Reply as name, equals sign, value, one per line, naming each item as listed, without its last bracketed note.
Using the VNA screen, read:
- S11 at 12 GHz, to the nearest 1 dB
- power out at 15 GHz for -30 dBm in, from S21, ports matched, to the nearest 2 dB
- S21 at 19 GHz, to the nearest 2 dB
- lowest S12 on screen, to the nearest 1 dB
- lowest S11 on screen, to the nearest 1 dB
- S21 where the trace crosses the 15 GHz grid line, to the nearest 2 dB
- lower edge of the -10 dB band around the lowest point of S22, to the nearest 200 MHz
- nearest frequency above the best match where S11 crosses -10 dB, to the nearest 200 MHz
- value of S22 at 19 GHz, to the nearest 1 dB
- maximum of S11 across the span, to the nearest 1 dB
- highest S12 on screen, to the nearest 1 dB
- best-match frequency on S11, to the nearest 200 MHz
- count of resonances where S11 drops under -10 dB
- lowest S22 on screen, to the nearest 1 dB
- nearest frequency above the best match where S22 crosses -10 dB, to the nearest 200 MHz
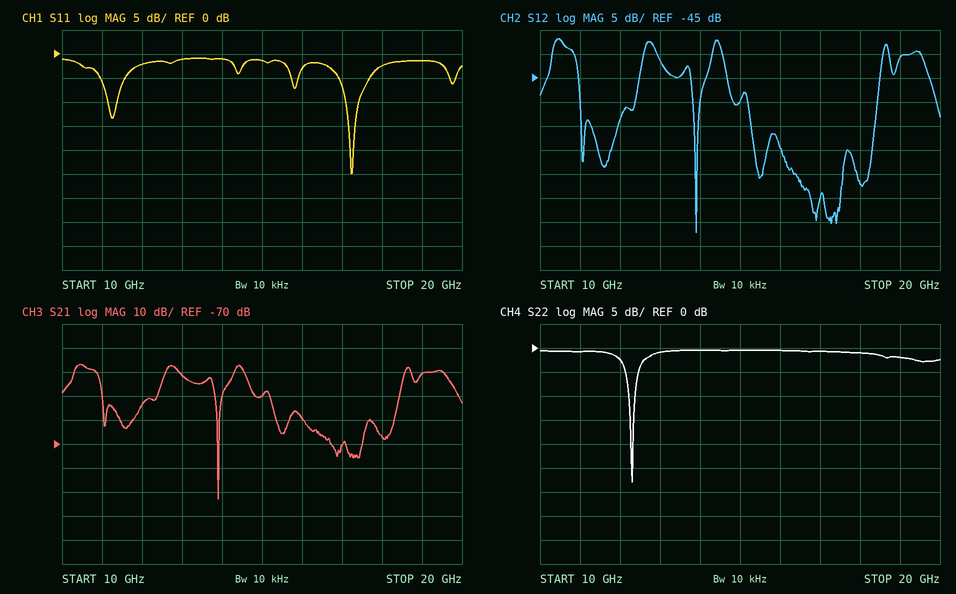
S11 at 12 GHz, to the nearest 1 dB = -2 dB
power out at 15 GHz for -30 dBm in, from S21, ports matched, to the nearest 2 dB = -80 dBm
S21 at 19 GHz, to the nearest 2 dB = -40 dB
lowest S12 on screen, to the nearest 1 dB = -77 dB
lowest S11 on screen, to the nearest 1 dB = -25 dB
S21 where the trace crosses the 15 GHz grid line, to the nearest 2 dB = -50 dB
lower edge of the -10 dB band around the lowest point of S22, to the nearest 200 MHz = 12.2 GHz
nearest frequency above the best match where S11 crosses -10 dB, to the nearest 200 MHz = 17.4 GHz
value of S22 at 19 GHz, to the nearest 1 dB = -2 dB
maximum of S11 across the span, to the nearest 1 dB = -1 dB
highest S12 on screen, to the nearest 1 dB = -37 dB
best-match frequency on S11, to the nearest 200 MHz = 17.2 GHz
count of resonances where S11 drops under -10 dB = 2
lowest S22 on screen, to the nearest 1 dB = -28 dB
nearest frequency above the best match where S22 crosses -10 dB, to the nearest 200 MHz = 12.4 GHz
